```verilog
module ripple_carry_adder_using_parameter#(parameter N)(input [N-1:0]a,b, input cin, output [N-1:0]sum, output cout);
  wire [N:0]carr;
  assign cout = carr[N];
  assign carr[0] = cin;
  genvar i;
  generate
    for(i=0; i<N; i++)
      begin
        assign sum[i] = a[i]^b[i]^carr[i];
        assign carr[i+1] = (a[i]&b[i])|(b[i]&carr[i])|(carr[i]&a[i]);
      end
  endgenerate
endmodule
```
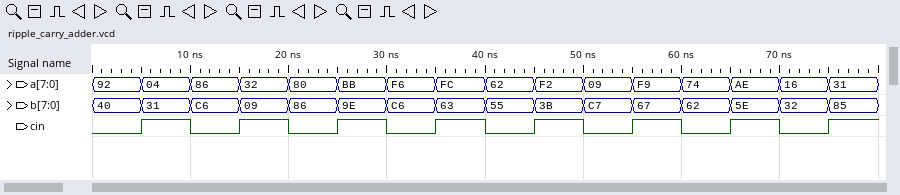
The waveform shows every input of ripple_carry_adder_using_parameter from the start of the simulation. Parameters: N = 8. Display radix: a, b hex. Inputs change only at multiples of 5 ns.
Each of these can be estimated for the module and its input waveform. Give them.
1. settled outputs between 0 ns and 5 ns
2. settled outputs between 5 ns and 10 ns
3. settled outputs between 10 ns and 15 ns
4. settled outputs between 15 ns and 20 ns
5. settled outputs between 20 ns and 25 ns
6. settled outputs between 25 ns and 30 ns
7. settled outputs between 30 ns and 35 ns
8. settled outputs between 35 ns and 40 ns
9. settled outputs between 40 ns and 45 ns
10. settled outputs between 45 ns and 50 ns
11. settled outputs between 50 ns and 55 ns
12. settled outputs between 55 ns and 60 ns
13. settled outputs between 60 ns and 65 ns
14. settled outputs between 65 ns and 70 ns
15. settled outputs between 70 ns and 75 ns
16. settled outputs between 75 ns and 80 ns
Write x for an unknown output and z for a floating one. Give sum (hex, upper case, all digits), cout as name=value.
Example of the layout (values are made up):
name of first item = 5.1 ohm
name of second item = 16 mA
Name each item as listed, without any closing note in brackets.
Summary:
settled outputs between 0 ns and 5 ns = sum=D2, cout=0
settled outputs between 5 ns and 10 ns = sum=36, cout=0
settled outputs between 10 ns and 15 ns = sum=4C, cout=1
settled outputs between 15 ns and 20 ns = sum=3C, cout=0
settled outputs between 20 ns and 25 ns = sum=06, cout=1
settled outputs between 25 ns and 30 ns = sum=5A, cout=1
settled outputs between 30 ns and 35 ns = sum=BC, cout=1
settled outputs between 35 ns and 40 ns = sum=60, cout=1
settled outputs between 40 ns and 45 ns = sum=B7, cout=0
settled outputs between 45 ns and 50 ns = sum=2E, cout=1
settled outputs between 50 ns and 55 ns = sum=D0, cout=0
settled outputs between 55 ns and 60 ns = sum=61, cout=1
settled outputs between 60 ns and 65 ns = sum=D6, cout=0
settled outputs between 65 ns and 70 ns = sum=0D, cout=1
settled outputs between 70 ns and 75 ns = sum=48, cout=0
settled outputs between 75 ns and 80 ns = sum=B7, cout=0
